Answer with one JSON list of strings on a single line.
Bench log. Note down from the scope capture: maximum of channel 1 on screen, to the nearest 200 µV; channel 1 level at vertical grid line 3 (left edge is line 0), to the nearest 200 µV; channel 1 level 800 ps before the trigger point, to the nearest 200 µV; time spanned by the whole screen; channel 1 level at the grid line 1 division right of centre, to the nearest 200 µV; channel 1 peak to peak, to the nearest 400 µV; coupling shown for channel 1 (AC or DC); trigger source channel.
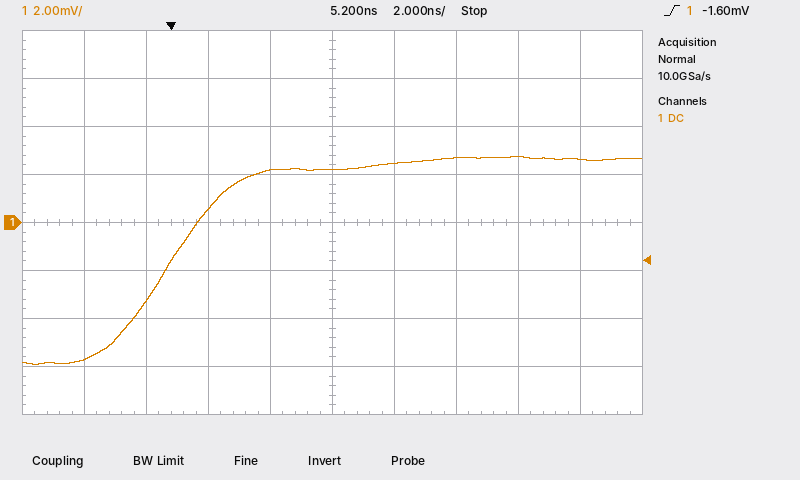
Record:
["2.8 mV", "600 µV", "-3.2 mV", "20 ns", "2.4 mV", "8.8 mV", "DC", "channel 1"]
